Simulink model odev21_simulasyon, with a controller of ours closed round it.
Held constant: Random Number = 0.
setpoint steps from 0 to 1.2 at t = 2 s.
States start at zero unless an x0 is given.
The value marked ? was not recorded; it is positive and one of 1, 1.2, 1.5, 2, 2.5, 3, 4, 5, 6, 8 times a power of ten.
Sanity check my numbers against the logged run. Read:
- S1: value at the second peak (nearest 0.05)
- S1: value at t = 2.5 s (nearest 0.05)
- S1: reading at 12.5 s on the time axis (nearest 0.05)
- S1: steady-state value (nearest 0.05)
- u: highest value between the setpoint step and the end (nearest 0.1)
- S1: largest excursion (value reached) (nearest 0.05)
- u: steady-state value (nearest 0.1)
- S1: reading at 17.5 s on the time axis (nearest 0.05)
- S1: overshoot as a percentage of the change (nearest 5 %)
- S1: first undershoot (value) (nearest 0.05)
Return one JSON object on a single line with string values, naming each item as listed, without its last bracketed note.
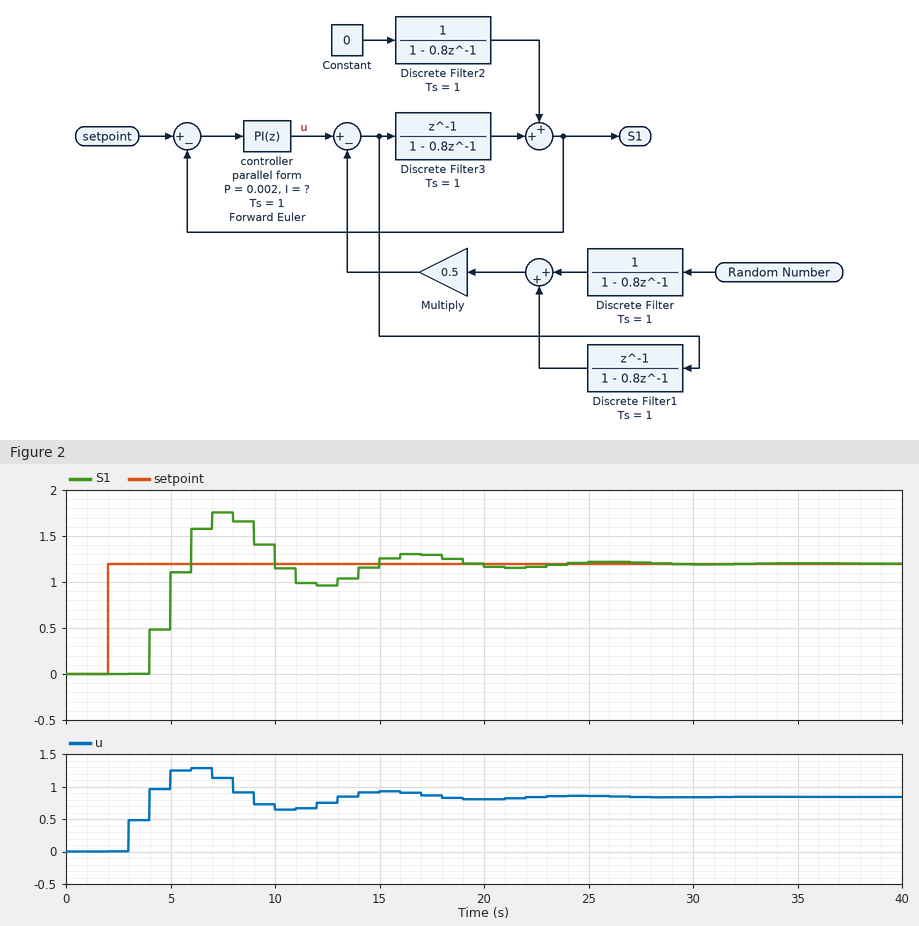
{"S1: value at the second peak": "1.30", "S1: value at t = 2.5 s": "0.00", "S1: reading at 12.5 s on the time axis": "0.95", "S1: steady-state value": "1.20", "u: highest value between the setpoint step and the end": "1.3", "S1: largest excursion (value reached)": "1.75", "u: steady-state value": "0.8", "S1: reading at 17.5 s on the time axis": "1.30", "S1: overshoot as a percentage of the change": "45 %", "S1: first undershoot (value)": "0.95"}
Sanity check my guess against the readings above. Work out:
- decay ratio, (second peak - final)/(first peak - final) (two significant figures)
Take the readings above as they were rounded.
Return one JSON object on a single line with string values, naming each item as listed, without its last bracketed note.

{"decay ratio, (second peak - final)/(first peak - final)": "0.18"}
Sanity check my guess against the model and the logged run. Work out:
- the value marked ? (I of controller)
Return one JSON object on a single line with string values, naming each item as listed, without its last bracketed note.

{"the value marked ?": "0.4"}
